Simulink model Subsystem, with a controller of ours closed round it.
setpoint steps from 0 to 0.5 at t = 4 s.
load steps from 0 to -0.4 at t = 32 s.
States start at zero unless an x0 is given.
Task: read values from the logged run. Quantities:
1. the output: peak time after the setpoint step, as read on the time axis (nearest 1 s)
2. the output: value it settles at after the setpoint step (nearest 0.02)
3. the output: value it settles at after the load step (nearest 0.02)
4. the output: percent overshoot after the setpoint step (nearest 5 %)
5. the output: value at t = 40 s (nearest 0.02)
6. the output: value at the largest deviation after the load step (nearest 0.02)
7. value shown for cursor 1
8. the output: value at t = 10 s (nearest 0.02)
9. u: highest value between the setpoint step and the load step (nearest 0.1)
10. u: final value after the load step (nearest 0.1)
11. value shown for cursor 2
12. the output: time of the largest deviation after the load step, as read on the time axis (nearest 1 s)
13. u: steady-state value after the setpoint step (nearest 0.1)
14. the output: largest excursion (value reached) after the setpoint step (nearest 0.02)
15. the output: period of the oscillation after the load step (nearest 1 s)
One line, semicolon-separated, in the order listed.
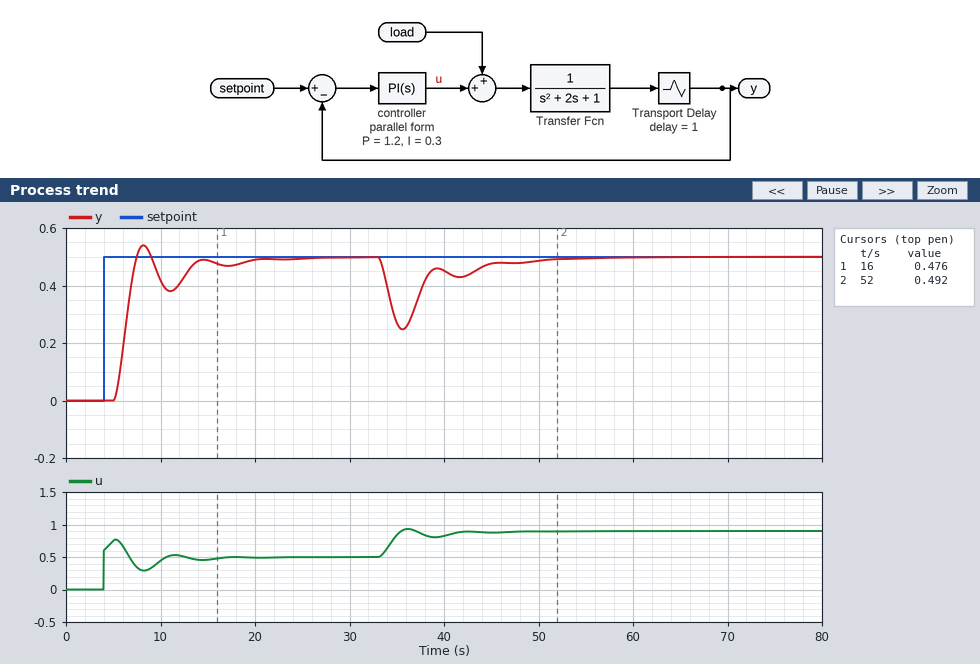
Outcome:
8 s; 0.50; 0.50; 10 %; 0.46; 0.24; 0.476; 0.42; 0.8; 0.9; 0.492; 36 s; 0.5; 0.54; 6 s
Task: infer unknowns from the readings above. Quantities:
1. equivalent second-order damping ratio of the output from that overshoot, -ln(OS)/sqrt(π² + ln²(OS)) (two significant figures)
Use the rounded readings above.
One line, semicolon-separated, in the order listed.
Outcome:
0.59
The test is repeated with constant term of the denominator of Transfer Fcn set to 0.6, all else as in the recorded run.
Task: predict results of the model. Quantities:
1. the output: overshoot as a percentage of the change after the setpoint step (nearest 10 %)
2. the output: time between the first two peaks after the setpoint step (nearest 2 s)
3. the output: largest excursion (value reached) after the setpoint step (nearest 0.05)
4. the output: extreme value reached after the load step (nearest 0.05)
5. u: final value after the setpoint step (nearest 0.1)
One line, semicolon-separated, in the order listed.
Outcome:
30 %; 8 s; 0.65; 0.20; 0.3
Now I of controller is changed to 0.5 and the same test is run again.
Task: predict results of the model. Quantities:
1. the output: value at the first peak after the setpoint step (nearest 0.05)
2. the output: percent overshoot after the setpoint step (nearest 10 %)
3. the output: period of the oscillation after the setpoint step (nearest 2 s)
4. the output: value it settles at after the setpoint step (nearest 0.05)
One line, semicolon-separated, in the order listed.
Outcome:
0.65; 30 %; 6 s; 0.50
